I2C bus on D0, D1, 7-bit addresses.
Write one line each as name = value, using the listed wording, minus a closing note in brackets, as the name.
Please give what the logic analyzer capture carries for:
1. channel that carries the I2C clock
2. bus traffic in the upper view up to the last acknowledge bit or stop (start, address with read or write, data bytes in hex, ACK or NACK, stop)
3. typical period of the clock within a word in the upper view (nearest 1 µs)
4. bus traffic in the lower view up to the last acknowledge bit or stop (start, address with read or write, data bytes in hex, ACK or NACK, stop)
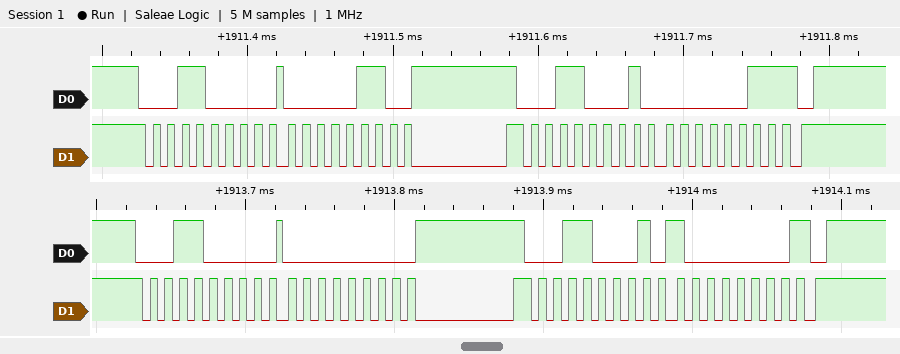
channel that carries the I2C clock = D1
bus traffic in the upper view up to the last acknowledge bit or stop = start, address 18 write ACK, 06 ACK, repeated start, address 18 read ACK, 03 NACK, stop
typical period of the clock within a word in the upper view = 10 µs
bus traffic in the lower view up to the last acknowledge bit or stop = start, address 18 write ACK, 00 ACK, repeated start, address 18 read ACK, 80 NACK, stop
